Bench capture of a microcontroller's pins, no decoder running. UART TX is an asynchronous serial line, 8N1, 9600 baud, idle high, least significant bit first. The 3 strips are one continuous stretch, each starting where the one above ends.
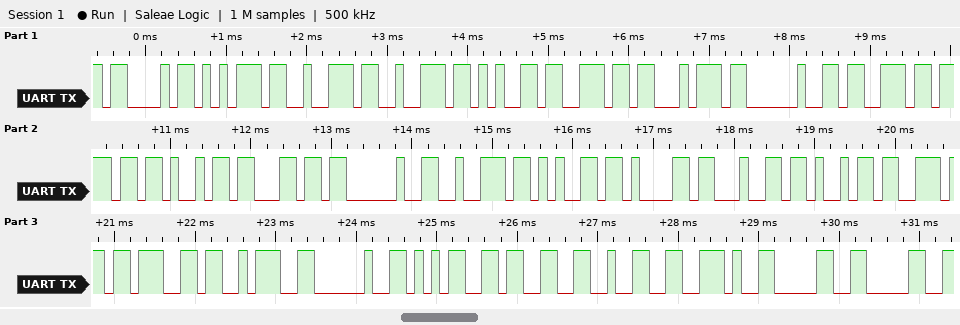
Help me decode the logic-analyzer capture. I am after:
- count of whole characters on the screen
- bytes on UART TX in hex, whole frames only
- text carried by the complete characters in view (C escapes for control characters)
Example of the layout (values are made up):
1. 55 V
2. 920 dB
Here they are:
1. 28
2. 43 75 72 72 65 6E 74 20 73 6F 69 6C 20 72 65 61 64 69 6E 67 3A 20 35 33 32 2E 30 30
3. "Current soil reading: 532.00"
